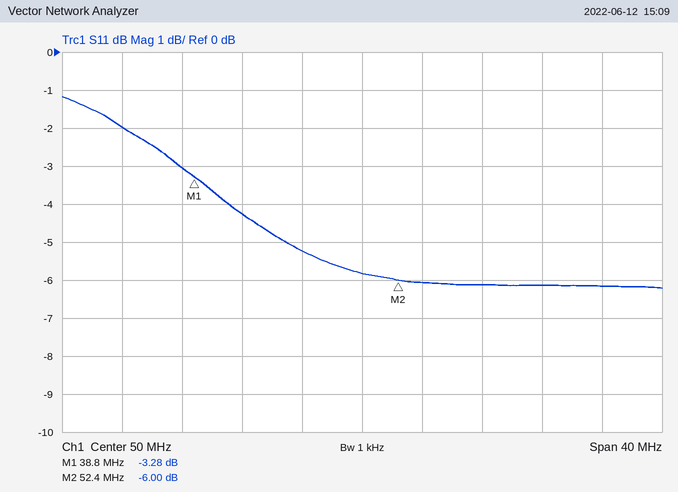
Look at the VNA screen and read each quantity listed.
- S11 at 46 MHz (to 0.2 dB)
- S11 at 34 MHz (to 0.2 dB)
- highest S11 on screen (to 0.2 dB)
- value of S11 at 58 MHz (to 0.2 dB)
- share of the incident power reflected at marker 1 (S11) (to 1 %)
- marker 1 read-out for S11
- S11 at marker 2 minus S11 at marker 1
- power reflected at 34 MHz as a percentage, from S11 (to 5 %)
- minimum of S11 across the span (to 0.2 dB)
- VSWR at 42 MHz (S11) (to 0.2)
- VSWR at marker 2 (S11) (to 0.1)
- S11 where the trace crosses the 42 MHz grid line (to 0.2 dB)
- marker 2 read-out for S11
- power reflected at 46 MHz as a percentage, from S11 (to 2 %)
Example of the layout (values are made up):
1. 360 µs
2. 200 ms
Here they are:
1. -5.2 dB
2. -2.0 dB
3. -1.2 dB
4. -6.2 dB
5. 47 %
6. -3.28 dB
7. -2.72 dB
8. 65 %
9. -6.2 dB
10. 4.2
11. 3.0
12. -4.2 dB
13. -6.00 dB
14. 30 %
